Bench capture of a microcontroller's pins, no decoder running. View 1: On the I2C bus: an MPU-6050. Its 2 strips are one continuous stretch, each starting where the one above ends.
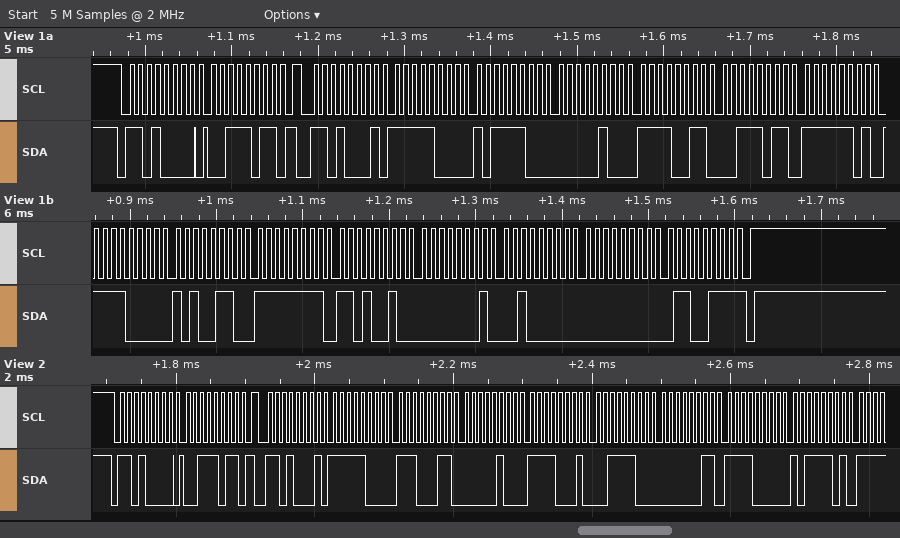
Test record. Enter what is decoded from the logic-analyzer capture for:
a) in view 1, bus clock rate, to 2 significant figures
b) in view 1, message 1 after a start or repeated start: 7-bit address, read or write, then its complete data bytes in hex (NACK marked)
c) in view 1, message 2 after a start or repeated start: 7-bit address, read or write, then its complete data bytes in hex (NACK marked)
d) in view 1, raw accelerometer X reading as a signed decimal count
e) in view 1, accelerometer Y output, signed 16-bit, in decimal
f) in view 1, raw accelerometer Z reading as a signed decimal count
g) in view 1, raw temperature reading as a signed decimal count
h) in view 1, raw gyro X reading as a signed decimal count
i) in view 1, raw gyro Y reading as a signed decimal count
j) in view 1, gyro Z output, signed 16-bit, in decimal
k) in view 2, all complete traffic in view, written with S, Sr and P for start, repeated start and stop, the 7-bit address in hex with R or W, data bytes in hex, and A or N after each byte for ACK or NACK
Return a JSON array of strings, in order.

["100 kHz", "0x68 write: 3B", "0x68 read: F8 BC 04 F3 3B FD F0 A6 FF D2 01 20 00 67 NACK", "-1860", "1267", "15357", "-3930", "-46", "288", "103", "S 68W A 3B A Sr 68R A F8 A E3 A 04 A F1 A 3C A 03 A F0 A BD A"]
